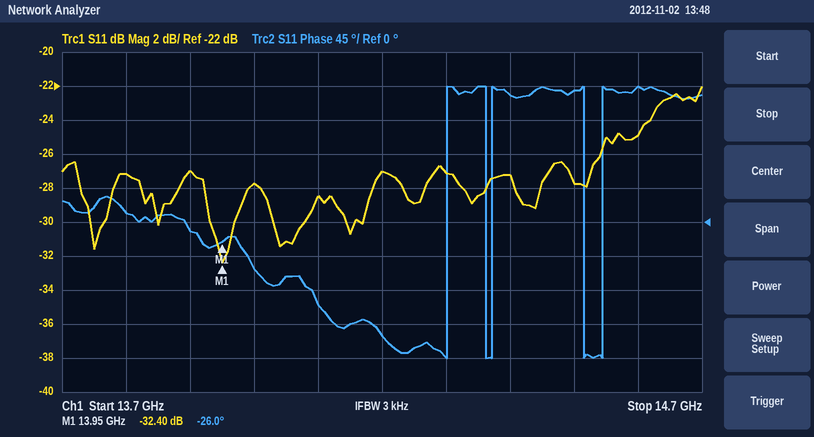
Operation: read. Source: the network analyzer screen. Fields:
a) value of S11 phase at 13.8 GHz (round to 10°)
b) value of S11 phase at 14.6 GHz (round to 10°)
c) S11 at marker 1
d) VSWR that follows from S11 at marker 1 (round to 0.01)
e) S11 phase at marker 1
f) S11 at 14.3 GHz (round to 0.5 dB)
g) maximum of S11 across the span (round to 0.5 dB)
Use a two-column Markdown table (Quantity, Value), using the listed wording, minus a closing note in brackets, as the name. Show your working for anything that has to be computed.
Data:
| Quantity | Value |
|---|---|
| value of S11 phase at 13.8 GHz | 10° |
| value of S11 phase at 14.6 GHz | 180° |
| S11 at marker 1 | -32.40 dB |
| VSWR that follows from S11 at marker 1 | (1 + 0.0240)/(1 − 0.0240) ≈ 1.05 |
| S11 phase at marker 1 | -26.0° |
| S11 at 14.3 GHz | -27.0 dB |
| maximum of S11 across the span | -22.0 dB |
